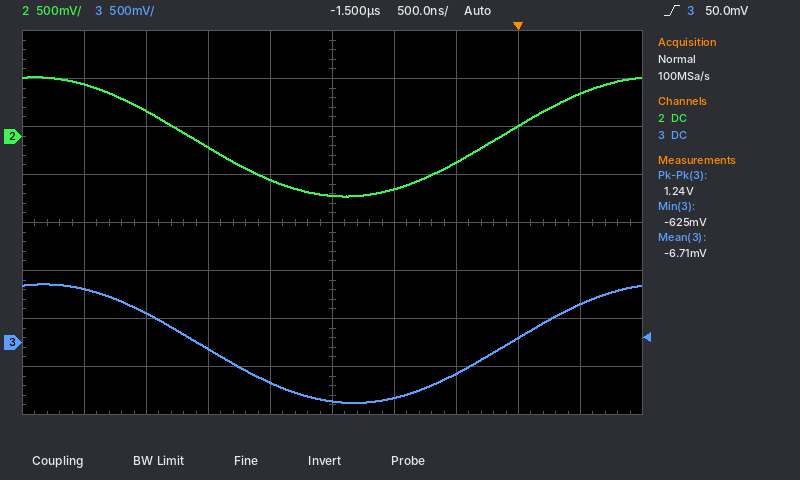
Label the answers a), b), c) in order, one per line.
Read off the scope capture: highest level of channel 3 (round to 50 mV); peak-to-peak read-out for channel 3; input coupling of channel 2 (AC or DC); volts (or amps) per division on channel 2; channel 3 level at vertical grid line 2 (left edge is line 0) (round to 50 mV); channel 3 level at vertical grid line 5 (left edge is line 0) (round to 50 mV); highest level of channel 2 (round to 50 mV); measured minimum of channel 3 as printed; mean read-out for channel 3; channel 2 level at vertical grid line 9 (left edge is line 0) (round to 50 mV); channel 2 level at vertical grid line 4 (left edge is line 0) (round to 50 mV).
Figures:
a) 600 mV
b) 1.24 V
c) DC
d) 500 mV
e) 300 mV
f) -600 mV
g) 600 mV
h) -625 mV
i) -6.71 mV
j) 450 mV
k) -450 mV
